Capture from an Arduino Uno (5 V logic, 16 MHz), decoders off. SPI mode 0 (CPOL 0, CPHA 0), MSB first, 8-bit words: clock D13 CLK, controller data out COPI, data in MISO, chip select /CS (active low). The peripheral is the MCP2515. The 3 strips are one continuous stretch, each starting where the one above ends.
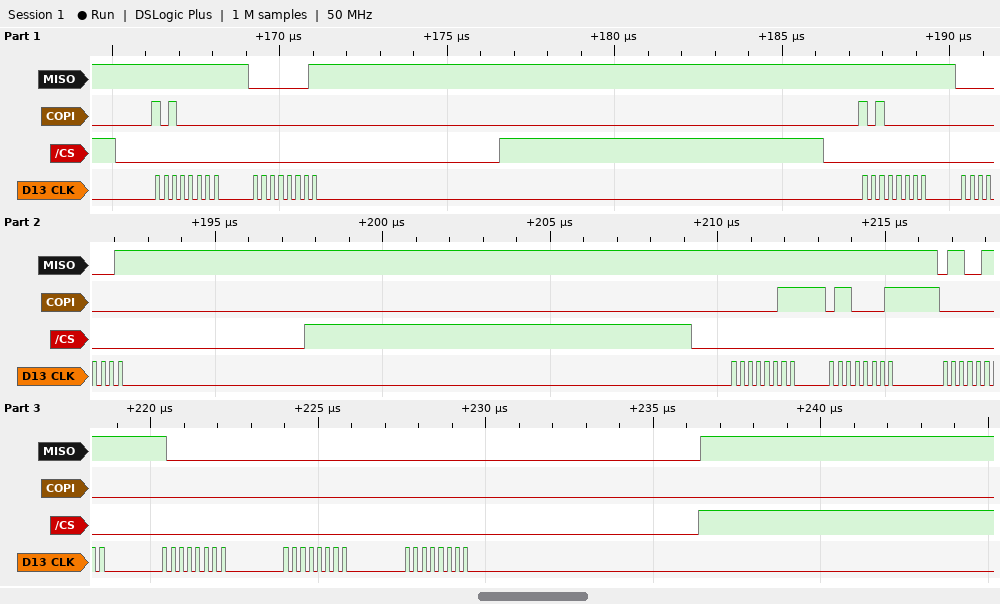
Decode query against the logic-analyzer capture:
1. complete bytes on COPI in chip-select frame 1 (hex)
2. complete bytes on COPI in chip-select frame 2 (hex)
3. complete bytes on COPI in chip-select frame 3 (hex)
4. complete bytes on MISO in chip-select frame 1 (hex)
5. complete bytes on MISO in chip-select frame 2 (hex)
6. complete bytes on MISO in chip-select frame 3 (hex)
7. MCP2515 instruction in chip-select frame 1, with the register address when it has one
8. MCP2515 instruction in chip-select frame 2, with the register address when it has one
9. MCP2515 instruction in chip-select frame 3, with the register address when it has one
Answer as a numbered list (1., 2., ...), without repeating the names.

1. 0xA0 0x00
2. 0xA0 0x00
3. 0x03 0x61 0x00 0x00 0x00 0x00
4. 0xFF 0x01
5. 0xFF 0x01
6. 0xFF 0xFF 0x67 0x80 0x00 0x00
7. READ STATUS
8. READ STATUS
9. READ 0x61
